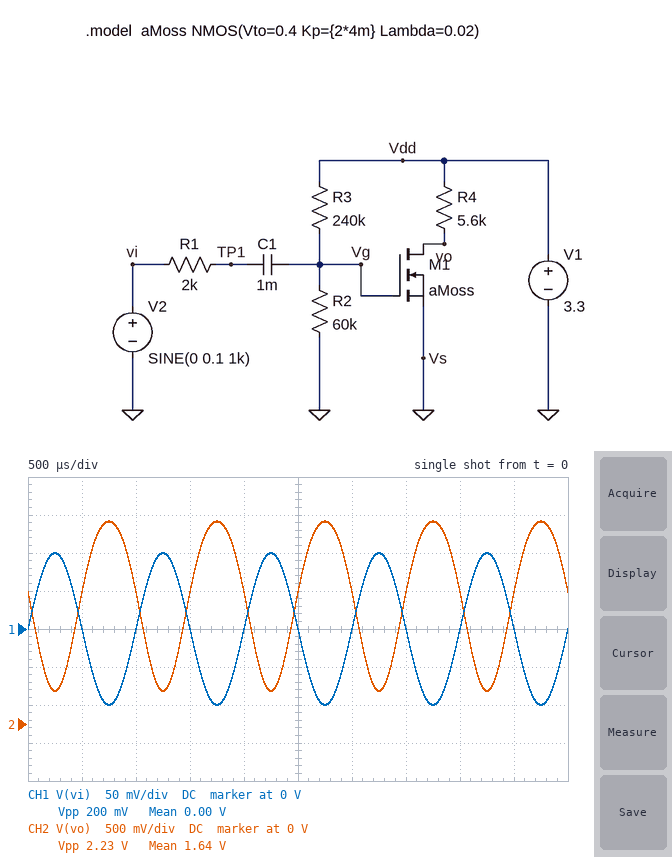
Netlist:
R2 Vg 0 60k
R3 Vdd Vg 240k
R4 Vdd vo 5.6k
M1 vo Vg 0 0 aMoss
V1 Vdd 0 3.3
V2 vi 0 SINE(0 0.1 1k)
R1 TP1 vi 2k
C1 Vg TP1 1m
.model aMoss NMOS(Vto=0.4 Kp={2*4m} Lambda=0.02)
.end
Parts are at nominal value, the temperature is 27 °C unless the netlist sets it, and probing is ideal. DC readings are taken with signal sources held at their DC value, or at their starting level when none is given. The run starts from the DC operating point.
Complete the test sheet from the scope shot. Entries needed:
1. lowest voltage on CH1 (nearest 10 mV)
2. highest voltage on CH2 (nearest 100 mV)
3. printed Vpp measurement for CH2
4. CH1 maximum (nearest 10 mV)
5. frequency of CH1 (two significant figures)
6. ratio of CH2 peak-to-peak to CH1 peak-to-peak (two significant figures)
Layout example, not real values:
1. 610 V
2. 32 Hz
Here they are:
1. -100 mV
2. 2.7 V
3. 2.23 V
4. 100 mV
5. 1.0 kHz
6. 11
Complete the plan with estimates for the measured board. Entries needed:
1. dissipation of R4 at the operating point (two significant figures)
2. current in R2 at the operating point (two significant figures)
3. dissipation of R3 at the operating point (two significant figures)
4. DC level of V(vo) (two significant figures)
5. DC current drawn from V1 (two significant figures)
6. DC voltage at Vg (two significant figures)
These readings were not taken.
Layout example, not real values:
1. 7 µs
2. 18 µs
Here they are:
1. 440 µW
2. 11 µA
3. 29 µW
4. 1.7 V
5. 290 µA
6. 660 mV
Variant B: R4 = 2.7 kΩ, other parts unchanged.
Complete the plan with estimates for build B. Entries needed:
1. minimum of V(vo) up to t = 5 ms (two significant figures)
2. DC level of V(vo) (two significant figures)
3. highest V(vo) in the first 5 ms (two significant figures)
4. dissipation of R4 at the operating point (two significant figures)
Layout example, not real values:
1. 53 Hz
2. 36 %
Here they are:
1. 1.9 V
2. 2.5 V
3. 3.0 V
4. 220 µW
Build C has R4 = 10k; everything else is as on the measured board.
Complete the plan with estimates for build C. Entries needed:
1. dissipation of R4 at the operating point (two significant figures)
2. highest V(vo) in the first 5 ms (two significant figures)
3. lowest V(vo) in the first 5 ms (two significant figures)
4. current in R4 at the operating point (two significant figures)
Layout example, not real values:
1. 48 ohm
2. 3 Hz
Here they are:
1. 750 µW
2. 2.2 V
3. 140 mV
4. 270 µA
